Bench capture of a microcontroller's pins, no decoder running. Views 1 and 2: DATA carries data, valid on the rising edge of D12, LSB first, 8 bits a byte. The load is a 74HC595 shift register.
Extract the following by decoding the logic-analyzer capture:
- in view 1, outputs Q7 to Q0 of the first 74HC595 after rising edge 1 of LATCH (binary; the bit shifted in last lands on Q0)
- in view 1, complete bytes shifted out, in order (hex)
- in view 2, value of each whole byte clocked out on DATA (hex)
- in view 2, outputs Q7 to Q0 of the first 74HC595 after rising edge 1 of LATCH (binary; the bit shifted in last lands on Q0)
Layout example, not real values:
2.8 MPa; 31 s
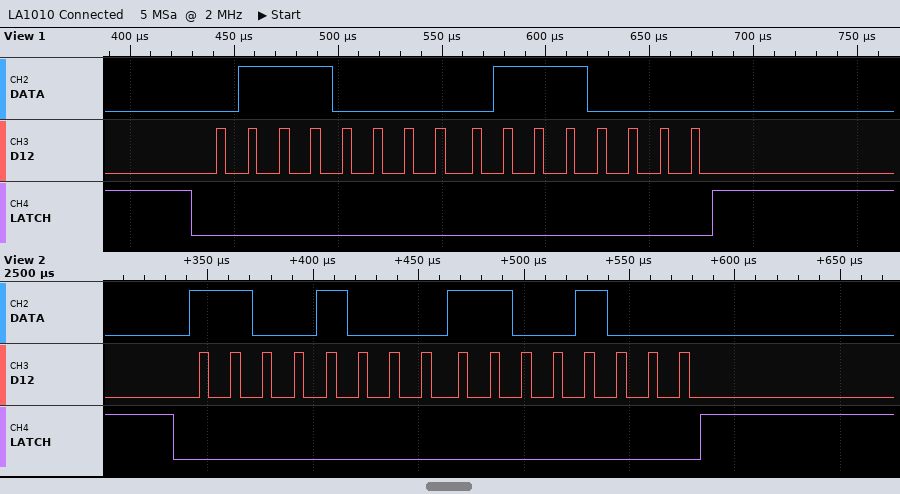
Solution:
01110000; 0E 0E; 0x13 0x13; 11001000
